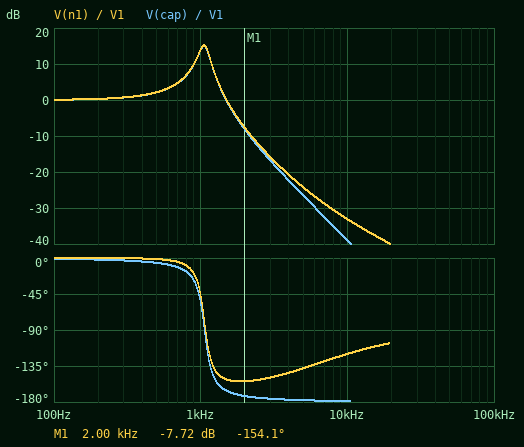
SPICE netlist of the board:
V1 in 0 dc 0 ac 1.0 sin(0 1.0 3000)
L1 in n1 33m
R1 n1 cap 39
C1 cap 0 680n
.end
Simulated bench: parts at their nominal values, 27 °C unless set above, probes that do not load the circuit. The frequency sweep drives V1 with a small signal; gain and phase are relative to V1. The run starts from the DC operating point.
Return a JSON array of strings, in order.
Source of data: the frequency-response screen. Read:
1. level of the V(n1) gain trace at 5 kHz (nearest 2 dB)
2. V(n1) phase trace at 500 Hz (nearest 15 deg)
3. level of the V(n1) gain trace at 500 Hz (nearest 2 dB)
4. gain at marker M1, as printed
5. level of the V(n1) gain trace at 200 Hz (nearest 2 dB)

["-24 dB", "0 deg", "2 dB", "-7.72 dB", "0 dB"]
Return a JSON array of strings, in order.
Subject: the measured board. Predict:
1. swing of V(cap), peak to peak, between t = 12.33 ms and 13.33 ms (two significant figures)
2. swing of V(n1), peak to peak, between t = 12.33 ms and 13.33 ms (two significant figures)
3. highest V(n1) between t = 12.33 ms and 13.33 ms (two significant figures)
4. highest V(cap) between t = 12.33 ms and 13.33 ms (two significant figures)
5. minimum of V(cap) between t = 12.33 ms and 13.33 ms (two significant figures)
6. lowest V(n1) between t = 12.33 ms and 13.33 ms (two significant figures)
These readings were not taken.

["290 mV", "320 mV", "160 mV", "140 mV", "-140 mV", "-160 mV"]
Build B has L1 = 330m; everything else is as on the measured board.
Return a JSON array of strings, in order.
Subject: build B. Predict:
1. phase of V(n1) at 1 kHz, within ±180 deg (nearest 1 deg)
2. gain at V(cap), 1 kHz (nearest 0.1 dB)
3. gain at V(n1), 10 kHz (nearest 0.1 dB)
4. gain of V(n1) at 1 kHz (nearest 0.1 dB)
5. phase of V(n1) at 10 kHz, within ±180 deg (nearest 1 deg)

["-169 deg", "-17.9 dB", "-53.2 dB", "-17.8 dB", "-121 deg"]
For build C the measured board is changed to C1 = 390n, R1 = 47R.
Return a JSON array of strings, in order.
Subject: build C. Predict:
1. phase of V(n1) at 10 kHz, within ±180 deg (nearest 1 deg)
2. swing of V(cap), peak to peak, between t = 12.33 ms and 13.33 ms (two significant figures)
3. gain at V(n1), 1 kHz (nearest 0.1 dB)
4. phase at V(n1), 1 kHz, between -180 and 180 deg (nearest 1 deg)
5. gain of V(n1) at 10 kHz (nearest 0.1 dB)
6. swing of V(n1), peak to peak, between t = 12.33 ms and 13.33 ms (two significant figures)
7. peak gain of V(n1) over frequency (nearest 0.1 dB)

["-130 deg", "560 mV", "6.0 dB", "-7 deg", "-30.3 dB", "590 mV", "16.0 dB"]
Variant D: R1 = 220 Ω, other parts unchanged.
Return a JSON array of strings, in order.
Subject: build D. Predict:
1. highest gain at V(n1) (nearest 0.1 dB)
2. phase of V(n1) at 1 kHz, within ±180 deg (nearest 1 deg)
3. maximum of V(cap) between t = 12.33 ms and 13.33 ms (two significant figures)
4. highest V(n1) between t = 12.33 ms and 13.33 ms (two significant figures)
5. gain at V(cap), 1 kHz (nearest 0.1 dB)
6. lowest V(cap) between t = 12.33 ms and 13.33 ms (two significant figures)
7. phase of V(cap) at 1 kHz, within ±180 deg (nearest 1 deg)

["3.3 dB", "-40 deg", "130 mV", "400 mV", "0.5 dB", "-130 mV", "-83 deg"]
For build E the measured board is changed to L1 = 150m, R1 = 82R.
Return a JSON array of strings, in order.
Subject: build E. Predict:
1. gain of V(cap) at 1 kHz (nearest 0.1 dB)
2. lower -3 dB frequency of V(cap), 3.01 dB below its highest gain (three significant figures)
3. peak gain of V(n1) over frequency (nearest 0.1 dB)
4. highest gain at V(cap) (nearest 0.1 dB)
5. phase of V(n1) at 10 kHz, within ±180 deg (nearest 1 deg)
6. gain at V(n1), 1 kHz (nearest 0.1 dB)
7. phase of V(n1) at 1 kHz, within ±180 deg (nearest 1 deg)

["-9.7 dB", "449 Hz", "15.3 dB", "15.2 dB", "-105 deg", "-9.2 dB", "-154 deg"]
